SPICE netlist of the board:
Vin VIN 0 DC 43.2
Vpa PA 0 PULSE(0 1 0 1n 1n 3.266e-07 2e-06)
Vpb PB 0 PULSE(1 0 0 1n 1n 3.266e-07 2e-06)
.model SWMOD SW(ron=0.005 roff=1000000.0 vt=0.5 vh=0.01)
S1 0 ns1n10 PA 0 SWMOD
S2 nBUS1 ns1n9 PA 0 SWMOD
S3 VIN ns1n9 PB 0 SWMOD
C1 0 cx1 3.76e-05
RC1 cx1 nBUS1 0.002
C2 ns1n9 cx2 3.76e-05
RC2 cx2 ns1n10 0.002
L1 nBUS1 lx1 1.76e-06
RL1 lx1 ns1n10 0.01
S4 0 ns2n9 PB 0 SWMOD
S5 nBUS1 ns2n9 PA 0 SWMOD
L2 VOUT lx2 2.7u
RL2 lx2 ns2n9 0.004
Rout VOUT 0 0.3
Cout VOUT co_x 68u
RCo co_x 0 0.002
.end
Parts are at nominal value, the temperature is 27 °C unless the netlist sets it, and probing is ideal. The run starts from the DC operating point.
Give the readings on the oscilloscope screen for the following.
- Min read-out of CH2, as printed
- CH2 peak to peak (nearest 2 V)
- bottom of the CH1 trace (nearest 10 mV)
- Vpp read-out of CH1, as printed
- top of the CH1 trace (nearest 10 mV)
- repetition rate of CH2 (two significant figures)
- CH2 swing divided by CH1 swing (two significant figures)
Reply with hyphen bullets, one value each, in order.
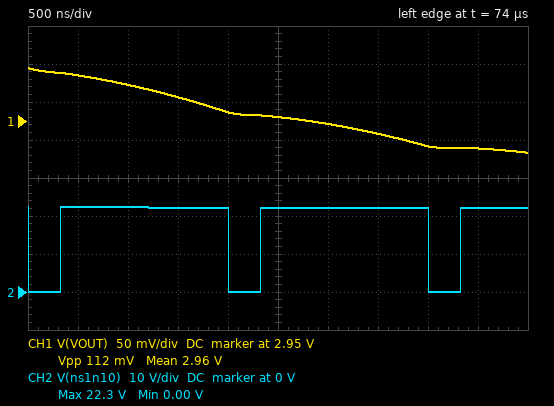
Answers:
- 0.00 V
- 22 V
- 2.91 V
- 112 mV
- 3.02 V
- 500 kHz
- 200
